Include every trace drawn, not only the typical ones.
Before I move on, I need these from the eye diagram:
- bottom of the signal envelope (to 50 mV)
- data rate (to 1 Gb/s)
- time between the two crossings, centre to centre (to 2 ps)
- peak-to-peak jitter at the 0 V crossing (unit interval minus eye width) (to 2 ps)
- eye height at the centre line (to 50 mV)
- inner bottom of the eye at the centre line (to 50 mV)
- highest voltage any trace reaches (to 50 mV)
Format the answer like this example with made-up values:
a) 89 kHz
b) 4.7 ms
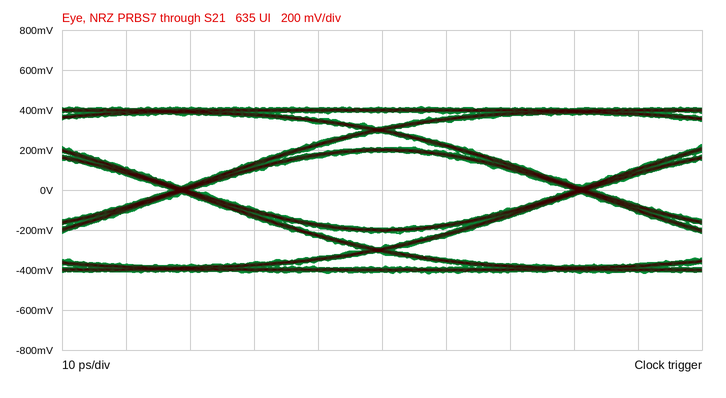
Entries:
a) -400 mV
b) 16 Gb/s
c) 62 ps
d) 4 ps
e) 400 mV
f) -200 mV
g) 400 mV
